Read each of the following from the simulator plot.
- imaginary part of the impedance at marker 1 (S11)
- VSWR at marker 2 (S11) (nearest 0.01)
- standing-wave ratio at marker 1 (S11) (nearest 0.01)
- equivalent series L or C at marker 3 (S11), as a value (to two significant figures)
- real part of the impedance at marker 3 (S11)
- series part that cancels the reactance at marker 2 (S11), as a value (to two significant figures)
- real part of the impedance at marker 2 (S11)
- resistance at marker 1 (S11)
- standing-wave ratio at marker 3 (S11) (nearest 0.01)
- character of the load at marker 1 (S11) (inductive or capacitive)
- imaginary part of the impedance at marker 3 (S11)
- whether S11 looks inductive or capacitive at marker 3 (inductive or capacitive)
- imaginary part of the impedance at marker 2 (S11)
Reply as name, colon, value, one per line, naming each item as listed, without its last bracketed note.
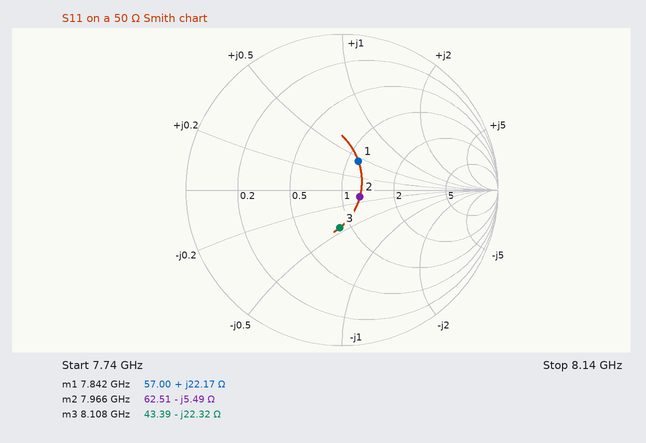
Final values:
imaginary part of the impedance at marker 1: +22.17 Ω
VSWR at marker 2 (S11): 1.28
standing-wave ratio at marker 1 (S11): 1.54
equivalent series L or C at marker 3 (S11), as a value: 880 fF
real part of the impedance at marker 3: 43.39 Ω
series part that cancels the reactance at marker 2 (S11), as a value: 110 pH
real part of the impedance at marker 2: 62.51 Ω
resistance at marker 1: 57.00 Ω
standing-wave ratio at marker 3 (S11): 1.64
character of the load at marker 1 (S11): inductive
imaginary part of the impedance at marker 3: -22.32 Ω
whether S11 looks inductive or capacitive at marker 3: capacitive
imaginary part of the impedance at marker 2: -5.49 Ω
